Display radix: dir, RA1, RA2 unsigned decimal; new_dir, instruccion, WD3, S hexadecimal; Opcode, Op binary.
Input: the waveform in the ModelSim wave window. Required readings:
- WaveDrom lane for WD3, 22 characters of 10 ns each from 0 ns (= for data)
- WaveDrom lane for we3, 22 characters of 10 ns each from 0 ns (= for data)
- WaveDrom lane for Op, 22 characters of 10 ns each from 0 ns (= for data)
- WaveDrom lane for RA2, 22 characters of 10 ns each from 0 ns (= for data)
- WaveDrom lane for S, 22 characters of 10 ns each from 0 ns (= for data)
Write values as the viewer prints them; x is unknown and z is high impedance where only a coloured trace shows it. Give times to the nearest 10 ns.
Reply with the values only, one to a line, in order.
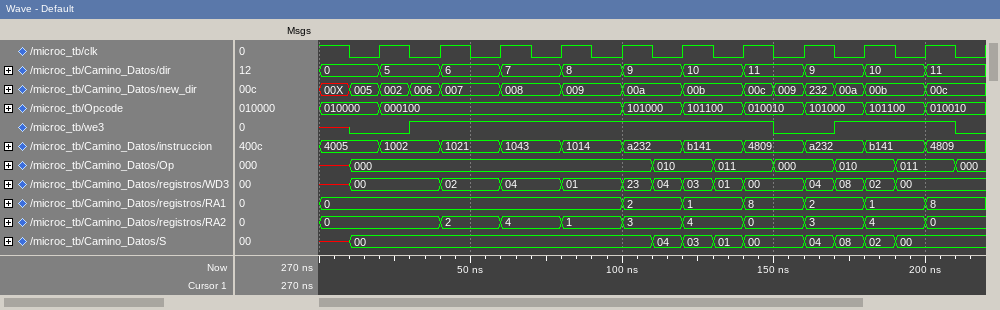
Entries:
{name: 'WD3', wave: 'x=..=.=.=.=====.====..', data: '00 02 04 01 23 04 03 01 00 04 08 02 00'}
{name: 'we3', wave: 'x0.1...........0.1...0'}
{name: 'Op', wave: 'x=.........=.=.=.=.=.=', data: '000 010 011 000 010 011 000'}
{name: 'RA2', wave: '=...=.=.=.=.=.=.=.=.=.', data: '0 2 4 1 3 4 0 3 4 0'}
{name: 'S', wave: 'x=.........====.====..', data: '00 04 03 01 00 04 08 02 00'}
